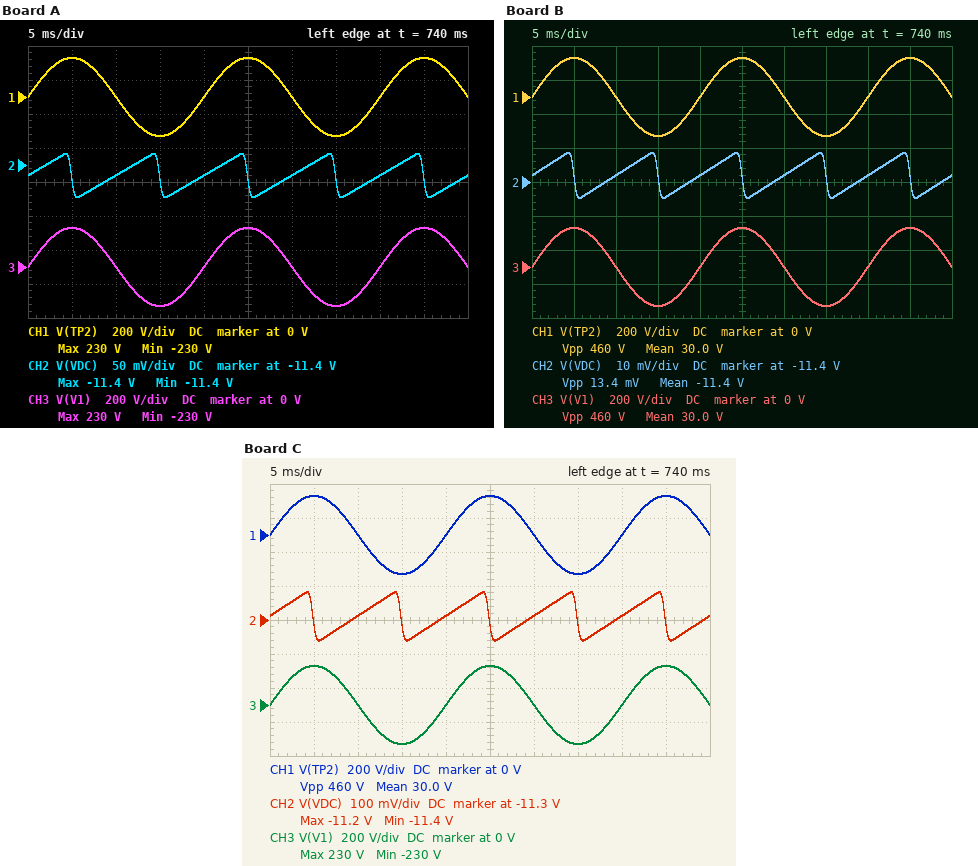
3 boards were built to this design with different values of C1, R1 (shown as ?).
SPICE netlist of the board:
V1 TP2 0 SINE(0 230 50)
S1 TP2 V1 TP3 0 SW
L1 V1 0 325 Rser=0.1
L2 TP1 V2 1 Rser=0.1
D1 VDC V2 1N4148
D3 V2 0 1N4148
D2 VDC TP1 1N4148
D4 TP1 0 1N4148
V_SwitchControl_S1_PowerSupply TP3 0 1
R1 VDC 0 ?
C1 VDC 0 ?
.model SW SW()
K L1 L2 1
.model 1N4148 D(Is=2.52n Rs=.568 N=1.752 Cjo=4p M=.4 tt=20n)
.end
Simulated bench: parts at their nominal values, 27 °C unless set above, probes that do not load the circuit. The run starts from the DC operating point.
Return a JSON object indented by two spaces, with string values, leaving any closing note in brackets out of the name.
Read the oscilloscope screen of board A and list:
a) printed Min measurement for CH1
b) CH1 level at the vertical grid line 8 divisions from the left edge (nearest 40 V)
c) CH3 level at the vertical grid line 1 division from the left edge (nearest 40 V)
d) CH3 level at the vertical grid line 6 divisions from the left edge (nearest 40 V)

{
  "printed Min measurement for CH1": "-230 V",
  "CH1 level at the vertical grid line 8 divisions from the left edge": "0 V",
  "CH3 level at the vertical grid line 1 division from the left edge": "240 V",
  "CH3 level at the vertical grid line 6 divisions from the left edge": "0 V"
}
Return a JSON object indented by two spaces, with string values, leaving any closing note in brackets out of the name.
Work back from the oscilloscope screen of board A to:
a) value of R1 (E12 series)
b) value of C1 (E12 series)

{
  "value of R1": "27 kΩ",
  "value of C1": "56 µF"
}
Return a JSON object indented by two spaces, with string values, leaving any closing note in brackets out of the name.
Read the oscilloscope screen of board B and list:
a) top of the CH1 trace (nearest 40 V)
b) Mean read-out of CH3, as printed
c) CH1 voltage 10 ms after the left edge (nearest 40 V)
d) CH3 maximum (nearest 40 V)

{
  "top of the CH1 trace": "240 V",
  "Mean read-out of CH3, as printed": "30.0 V",
  "CH1 voltage 10 ms after the left edge": "0 V",
  "CH3 maximum": "240 V"
}
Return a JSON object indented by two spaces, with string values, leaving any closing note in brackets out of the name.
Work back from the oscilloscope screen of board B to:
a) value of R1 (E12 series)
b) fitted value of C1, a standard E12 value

{
  "value of R1": "22 kΩ",
  "fitted value of C1, a standard E12 value": "330 µF"
}
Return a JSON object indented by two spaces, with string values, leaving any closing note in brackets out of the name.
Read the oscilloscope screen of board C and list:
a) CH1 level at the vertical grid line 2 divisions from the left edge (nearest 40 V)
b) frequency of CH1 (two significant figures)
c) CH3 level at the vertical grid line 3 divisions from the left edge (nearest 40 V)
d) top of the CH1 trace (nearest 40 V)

{
  "CH1 level at the vertical grid line 2 divisions from the left edge": "0 V",
  "frequency of CH1": "50 Hz",
  "CH3 level at the vertical grid line 3 divisions from the left edge": "-240 V",
  "top of the CH1 trace": "240 V"
}
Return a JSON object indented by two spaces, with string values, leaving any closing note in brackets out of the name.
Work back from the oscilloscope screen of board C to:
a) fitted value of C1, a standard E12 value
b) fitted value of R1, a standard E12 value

{
  "fitted value of C1, a standard E12 value": "82 µF",
  "fitted value of R1, a standard E12 value": "8.2 kΩ"
}
